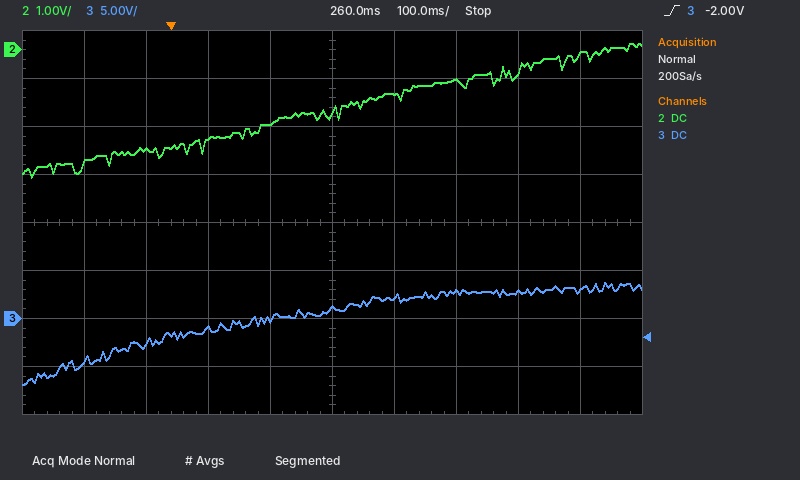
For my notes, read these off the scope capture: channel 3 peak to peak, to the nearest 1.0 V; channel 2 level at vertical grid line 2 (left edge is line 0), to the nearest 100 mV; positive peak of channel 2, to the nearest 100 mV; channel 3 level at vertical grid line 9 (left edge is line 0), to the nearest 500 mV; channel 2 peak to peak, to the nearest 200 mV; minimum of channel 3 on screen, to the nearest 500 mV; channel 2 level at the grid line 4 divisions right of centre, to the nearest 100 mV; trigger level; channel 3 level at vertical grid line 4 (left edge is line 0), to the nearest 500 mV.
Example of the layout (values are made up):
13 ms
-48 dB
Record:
11.0 V
-2.1 V
100 mV
3.0 V
2.8 V
-7.0 V
-100 mV
-2.00 V
0.0 V
